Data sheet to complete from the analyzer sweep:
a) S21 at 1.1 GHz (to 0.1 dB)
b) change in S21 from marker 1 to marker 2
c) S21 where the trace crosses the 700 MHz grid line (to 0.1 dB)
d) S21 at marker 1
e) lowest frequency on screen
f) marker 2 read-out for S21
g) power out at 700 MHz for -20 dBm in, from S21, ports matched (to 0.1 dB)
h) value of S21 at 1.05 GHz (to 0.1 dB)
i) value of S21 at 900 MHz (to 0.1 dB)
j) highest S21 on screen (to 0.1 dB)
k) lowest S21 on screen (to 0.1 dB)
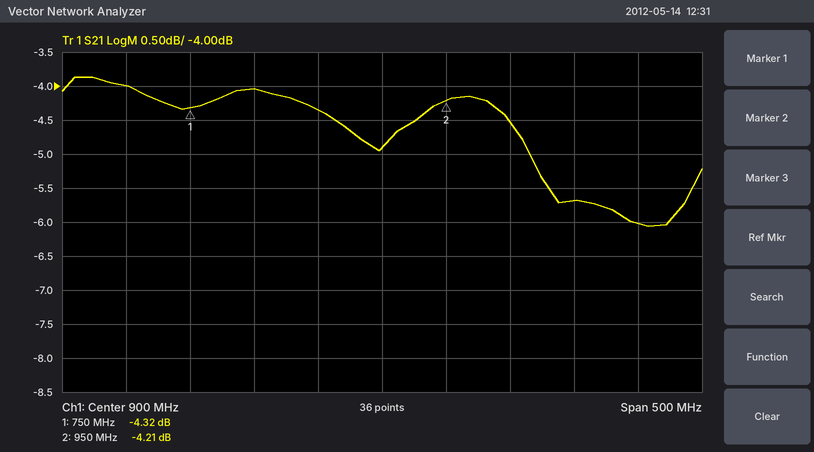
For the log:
-6.0 dB
0.11 dB
-4.0 dB
-4.32 dB
650 MHz
-4.21 dB
-24.0 dBm
-5.7 dB
-4.9 dB
-3.9 dB
-6.1 dB
